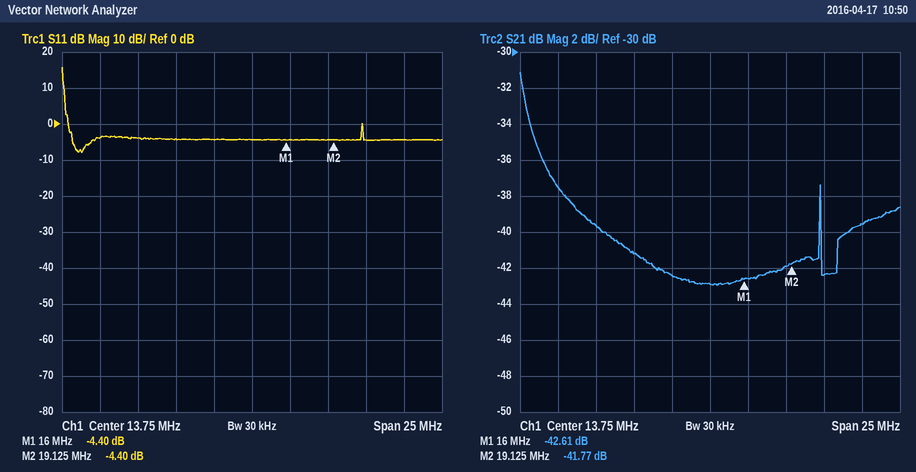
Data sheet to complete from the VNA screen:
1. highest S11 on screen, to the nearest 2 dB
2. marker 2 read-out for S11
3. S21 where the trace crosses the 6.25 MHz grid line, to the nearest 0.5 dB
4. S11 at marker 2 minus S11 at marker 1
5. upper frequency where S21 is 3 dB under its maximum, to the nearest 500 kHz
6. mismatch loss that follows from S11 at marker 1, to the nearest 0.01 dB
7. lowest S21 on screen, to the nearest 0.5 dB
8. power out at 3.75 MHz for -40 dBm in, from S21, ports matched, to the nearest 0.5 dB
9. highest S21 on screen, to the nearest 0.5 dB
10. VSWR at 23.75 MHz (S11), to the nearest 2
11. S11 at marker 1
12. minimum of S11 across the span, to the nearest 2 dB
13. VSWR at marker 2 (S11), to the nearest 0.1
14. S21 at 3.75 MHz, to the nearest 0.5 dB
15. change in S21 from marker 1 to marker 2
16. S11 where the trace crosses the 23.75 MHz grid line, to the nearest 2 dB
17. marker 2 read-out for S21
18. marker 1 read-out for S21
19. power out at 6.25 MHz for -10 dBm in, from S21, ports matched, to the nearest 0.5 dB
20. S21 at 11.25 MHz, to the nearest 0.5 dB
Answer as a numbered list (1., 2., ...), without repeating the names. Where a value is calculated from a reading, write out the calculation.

1. 16 dB
2. -4.40 dB
3. -39.5 dB
4. -4.4 − (-4.4) = 0.00 dB
5. 2.0 MHz
6. −10 log10(1 − 10^(-4.4/10)) ≈ 1.96 dB
7. -43.0 dB
8. -40 dBm + (-37.5 dB) = -77.5 dBm
9. -31.0 dB
10. |Γ| = 10^(-4/20) = 0.6310; VSWR = (1 + 0.6310)/(1 − 0.6310) ≈ 4
11. -4.40 dB
12. -8 dB
13. (1 + 0.6026)/(1 − 0.6026) ≈ 4.0
14. -37.5 dB
15. -41.77 − (-42.61) = 0.84 dB
16. -4 dB
17. -41.77 dB
18. -42.61 dB
19. -10 dBm + (-39.5 dB) = -49.5 dBm
20. -42.5 dB
